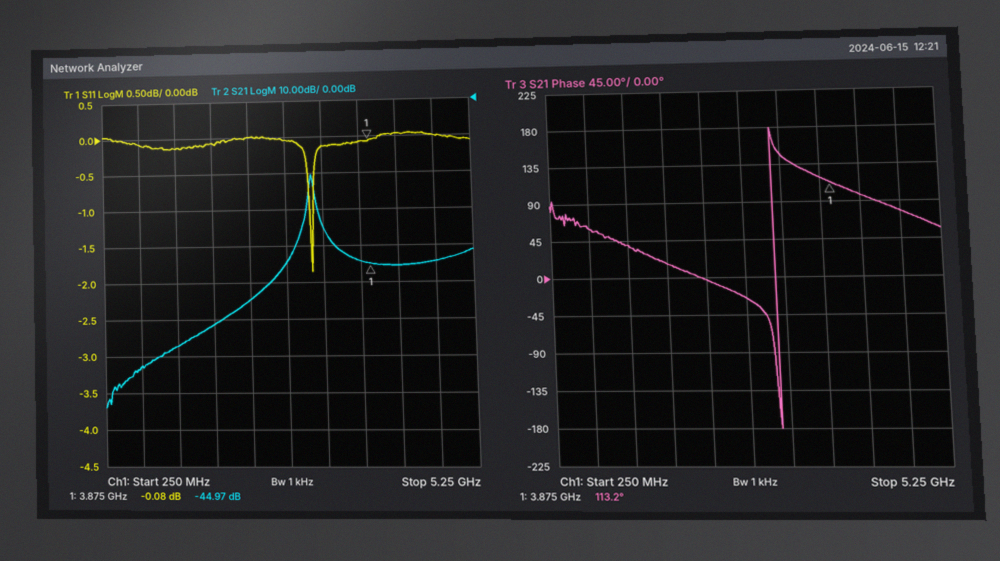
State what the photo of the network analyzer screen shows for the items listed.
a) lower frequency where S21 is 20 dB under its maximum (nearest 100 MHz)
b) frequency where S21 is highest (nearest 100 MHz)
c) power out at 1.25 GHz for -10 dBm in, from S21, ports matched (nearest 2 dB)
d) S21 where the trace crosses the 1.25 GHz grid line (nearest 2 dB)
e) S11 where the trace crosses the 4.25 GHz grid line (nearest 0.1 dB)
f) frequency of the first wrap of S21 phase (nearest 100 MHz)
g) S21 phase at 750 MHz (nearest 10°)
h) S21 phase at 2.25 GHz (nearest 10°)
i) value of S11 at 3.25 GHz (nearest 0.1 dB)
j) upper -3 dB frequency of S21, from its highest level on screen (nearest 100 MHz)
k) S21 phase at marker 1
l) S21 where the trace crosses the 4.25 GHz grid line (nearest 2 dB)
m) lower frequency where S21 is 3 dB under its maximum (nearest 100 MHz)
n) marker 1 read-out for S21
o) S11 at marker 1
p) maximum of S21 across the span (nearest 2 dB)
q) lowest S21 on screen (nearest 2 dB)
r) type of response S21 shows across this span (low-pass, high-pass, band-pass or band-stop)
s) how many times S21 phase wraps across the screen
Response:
2.9 GHz
3.1 GHz
-78 dBm
-68 dB
0.0 dB
3.1 GHz
60°
0°
-0.1 dB
3.1 GHz
113.2°
-46 dB
3.1 GHz
-44.97 dB
-0.08 dB
-20 dB
-84 dB
band-pass
1
